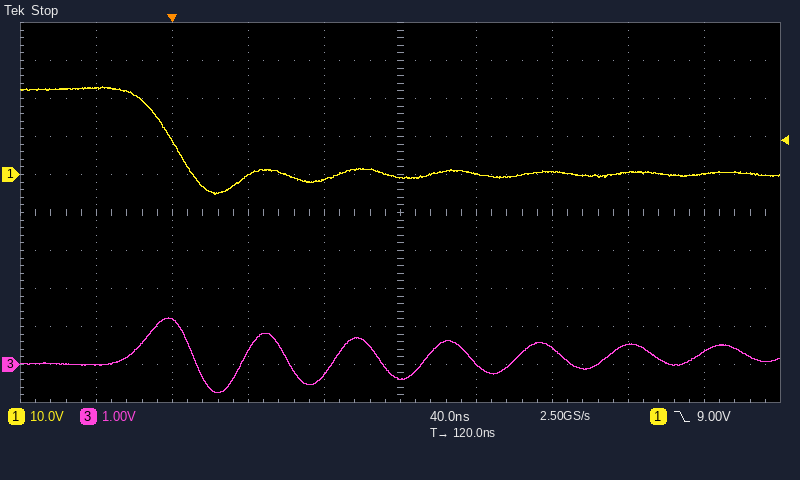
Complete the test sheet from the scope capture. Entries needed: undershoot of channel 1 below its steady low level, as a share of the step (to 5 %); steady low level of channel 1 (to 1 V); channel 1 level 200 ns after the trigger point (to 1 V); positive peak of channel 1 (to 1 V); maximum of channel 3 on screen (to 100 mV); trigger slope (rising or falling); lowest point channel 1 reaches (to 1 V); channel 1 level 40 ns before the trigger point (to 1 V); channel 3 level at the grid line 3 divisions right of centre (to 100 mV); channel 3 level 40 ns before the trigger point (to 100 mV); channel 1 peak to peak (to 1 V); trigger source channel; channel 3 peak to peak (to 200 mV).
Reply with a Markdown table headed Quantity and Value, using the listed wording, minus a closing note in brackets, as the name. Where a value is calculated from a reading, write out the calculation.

| Quantity | Value |
|---|---|
| undershoot of channel 1 below its steady low level, as a share of the step | 25 % |
| steady low level of channel 1 | 0 V |
| channel 1 level 200 ns after the trigger point | 1 V |
| positive peak of channel 1 | 23 V |
| maximum of channel 3 on screen | 1.2 V |
| trigger slope | falling |
| lowest point channel 1 reaches | -5 V |
| channel 1 level 40 ns before the trigger point | 23 V |
| channel 3 level at the grid line 3 divisions right of centre | 500 mV |
| channel 3 level 40 ns before the trigger point | 0.0 V |
| channel 1 peak to peak | 23 V − (-5 V) = 28 V |
| trigger source channel | channel 1 |
| channel 3 peak to peak | 2.0 V |
